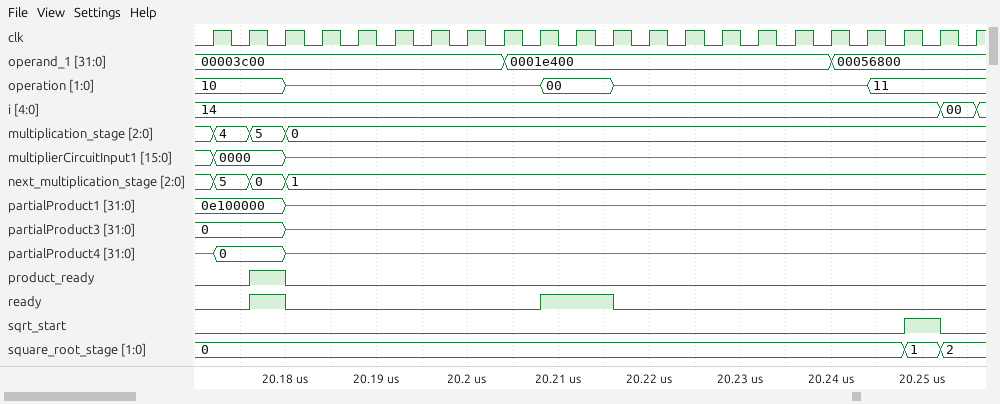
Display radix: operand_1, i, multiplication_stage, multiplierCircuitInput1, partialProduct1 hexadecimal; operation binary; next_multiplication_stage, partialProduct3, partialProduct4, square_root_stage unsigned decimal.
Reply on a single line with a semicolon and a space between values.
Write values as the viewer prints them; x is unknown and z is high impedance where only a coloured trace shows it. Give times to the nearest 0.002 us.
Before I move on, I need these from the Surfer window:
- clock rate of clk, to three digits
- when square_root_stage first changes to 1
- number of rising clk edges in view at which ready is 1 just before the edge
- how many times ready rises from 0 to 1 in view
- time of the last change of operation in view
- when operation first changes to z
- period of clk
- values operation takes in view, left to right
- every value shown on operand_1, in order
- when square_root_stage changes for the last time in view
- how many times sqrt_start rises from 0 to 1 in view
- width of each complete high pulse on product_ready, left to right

250 MHz; 20.248 us; 3; 2; 20.244 us; 20.18 us; 0.004 us; 10, z, 00, z, 11; 00003c00, 0001e400, 00056800; 20.252 us; 1; 0.004 us
